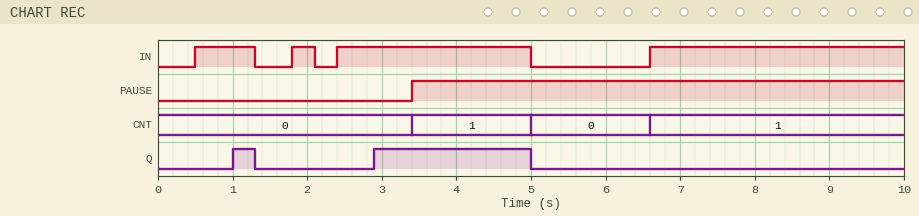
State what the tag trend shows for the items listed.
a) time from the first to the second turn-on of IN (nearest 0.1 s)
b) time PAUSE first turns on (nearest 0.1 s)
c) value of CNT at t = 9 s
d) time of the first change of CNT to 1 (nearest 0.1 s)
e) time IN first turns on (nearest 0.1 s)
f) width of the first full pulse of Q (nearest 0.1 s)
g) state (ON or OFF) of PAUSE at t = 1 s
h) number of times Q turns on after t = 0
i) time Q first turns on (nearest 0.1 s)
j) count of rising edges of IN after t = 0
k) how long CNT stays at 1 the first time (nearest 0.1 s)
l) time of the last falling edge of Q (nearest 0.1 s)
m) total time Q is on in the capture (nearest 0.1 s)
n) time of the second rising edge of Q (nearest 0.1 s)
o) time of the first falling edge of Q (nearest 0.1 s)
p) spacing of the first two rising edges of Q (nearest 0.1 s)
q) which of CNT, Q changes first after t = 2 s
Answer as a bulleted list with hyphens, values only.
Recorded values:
- 1.3 s
- 3.4 s
- 1
- 3.4 s
- 0.5 s
- 0.3 s
- OFF
- 2
- 1.0 s
- 4
- 1.6 s
- 5.0 s
- 2.4 s
- 2.9 s
- 1.3 s
- 1.9 s
- Q
